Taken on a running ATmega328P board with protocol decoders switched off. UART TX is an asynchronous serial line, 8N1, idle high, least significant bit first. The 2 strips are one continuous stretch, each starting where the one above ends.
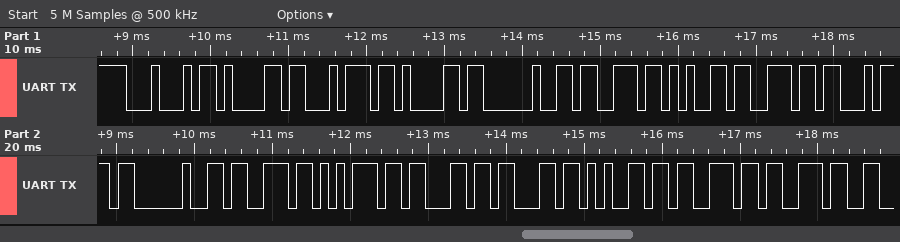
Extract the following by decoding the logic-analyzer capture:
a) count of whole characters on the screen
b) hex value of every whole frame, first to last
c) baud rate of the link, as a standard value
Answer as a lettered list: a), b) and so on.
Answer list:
a) 17
b) 44 61 74 61 20 73 65 6E 74 20 73 75 63 63 65 73 73
c) 9600 baud
